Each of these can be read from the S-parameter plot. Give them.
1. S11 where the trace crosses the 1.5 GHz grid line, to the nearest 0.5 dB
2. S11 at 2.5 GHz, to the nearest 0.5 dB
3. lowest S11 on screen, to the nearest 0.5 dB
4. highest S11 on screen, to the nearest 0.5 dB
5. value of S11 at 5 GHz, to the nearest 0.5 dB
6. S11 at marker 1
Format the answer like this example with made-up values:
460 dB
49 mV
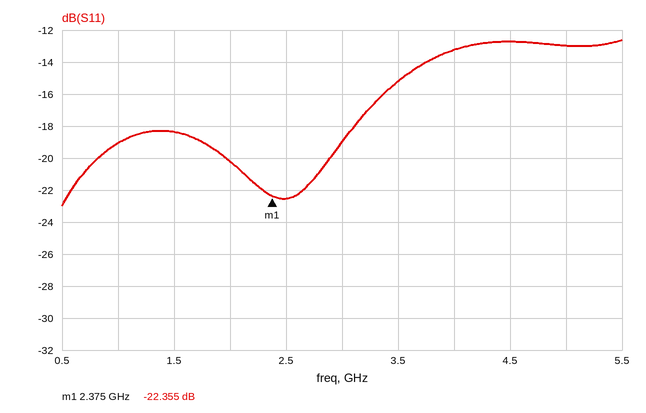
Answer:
-18.5 dB
-22.5 dB
-23.0 dB
-12.5 dB
-13.0 dB
-22.355 dB
